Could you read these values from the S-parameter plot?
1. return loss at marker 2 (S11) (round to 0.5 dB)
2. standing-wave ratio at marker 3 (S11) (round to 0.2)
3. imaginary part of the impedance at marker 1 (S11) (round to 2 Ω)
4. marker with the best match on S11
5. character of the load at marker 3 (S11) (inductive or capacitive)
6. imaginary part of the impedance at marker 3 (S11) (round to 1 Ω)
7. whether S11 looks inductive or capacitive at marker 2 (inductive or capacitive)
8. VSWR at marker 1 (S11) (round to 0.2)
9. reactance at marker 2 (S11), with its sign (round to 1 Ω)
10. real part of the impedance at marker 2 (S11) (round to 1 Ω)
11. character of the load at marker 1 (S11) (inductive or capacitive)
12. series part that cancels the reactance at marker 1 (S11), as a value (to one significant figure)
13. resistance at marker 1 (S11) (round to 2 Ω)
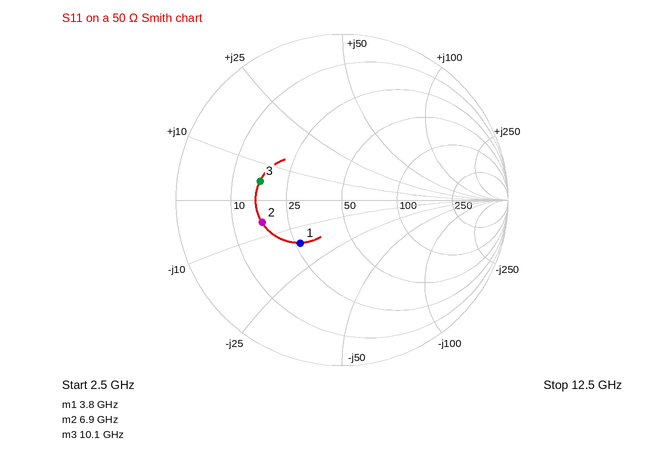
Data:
6.0 dB
3.0
-16 Ω
marker 1
inductive
+5 Ω
capacitive
2.2
-6 Ω
17 Ω
capacitive
700 pH
26 Ω
